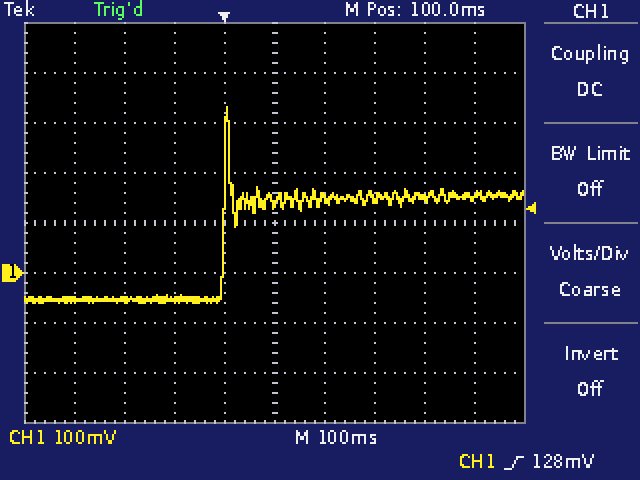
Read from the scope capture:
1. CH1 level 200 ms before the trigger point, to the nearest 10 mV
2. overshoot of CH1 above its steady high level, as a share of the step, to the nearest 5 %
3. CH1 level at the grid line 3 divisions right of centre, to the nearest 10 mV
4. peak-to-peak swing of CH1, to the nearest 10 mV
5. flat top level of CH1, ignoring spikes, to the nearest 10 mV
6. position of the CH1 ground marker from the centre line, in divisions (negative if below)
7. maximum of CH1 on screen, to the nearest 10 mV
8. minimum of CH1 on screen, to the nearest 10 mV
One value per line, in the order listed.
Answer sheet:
-50 mV
85 %
150 mV
390 mV
150 mV
-1.0 div
330 mV
-60 mV
